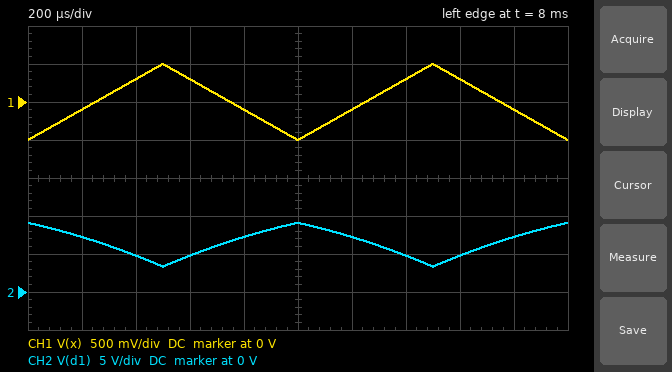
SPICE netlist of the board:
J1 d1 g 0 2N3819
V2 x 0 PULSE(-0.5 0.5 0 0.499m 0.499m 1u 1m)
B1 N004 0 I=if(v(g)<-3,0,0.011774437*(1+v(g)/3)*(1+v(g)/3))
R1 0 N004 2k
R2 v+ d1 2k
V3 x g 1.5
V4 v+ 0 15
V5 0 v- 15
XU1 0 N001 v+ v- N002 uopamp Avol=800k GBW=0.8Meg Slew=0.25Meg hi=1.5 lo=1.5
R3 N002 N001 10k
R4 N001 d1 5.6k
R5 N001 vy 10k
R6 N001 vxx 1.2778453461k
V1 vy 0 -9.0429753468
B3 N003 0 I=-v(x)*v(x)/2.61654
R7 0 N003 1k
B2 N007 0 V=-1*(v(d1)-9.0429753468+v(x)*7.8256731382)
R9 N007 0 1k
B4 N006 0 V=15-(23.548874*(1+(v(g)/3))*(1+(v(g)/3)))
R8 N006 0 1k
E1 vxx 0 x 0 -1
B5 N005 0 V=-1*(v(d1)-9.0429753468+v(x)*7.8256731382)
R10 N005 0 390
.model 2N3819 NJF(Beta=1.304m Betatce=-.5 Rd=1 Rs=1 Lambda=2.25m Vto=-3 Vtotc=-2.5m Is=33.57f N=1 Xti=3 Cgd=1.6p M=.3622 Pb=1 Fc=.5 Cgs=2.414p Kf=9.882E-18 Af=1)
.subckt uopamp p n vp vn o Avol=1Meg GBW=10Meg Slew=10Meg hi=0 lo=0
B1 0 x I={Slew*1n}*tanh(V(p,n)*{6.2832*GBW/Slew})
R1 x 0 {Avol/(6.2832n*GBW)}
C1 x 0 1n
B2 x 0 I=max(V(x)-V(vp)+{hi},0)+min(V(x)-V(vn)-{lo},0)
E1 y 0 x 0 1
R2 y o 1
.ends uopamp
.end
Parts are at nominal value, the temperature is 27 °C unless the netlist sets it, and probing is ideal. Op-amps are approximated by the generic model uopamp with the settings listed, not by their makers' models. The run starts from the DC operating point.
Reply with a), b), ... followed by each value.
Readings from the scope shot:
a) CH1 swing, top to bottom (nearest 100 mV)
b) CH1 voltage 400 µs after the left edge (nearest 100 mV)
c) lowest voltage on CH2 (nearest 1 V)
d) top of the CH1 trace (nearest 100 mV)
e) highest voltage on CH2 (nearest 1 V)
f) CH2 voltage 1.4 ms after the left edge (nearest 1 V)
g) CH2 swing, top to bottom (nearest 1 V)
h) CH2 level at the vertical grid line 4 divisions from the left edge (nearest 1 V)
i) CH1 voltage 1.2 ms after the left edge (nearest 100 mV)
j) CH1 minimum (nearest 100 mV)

a) 1.0 V
b) 300 mV
c) 3 V
d) 500 mV
e) 9 V
f) 5 V
g) 6 V
h) 7 V
i) -100 mV
j) -500 mV
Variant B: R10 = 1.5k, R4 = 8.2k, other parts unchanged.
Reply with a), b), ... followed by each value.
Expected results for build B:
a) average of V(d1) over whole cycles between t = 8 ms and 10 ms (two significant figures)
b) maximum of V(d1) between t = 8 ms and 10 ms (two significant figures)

a) 7.1 V
b) 9.9 V
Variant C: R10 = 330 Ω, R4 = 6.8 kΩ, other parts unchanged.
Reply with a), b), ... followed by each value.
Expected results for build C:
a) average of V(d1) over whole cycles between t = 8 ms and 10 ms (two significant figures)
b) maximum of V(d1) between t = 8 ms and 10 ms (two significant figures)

a) 6.8 V
b) 9.5 V
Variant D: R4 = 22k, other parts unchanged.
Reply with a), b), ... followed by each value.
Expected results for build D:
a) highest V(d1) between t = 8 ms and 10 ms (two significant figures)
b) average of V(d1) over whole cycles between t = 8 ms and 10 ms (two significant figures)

a) 11 V
b) 8.1 V
